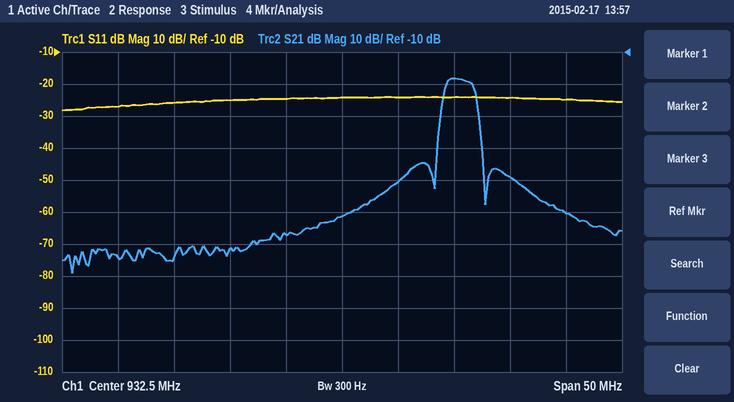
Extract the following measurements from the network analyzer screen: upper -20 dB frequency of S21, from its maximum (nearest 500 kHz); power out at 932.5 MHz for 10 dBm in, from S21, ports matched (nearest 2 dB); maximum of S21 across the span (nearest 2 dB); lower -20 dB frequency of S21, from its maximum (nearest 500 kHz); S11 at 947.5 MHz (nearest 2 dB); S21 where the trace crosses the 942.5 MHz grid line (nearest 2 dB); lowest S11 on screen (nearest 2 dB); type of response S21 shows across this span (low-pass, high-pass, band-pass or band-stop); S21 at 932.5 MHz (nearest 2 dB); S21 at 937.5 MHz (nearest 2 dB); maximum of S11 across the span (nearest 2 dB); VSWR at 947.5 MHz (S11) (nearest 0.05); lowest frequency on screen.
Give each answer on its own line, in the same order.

945.0 MHz
-52 dBm
-18 dB
941.0 MHz
-24 dB
-18 dB
-28 dB
band-pass
-62 dB
-50 dB
-24 dB
1.15
907.5 MHz
